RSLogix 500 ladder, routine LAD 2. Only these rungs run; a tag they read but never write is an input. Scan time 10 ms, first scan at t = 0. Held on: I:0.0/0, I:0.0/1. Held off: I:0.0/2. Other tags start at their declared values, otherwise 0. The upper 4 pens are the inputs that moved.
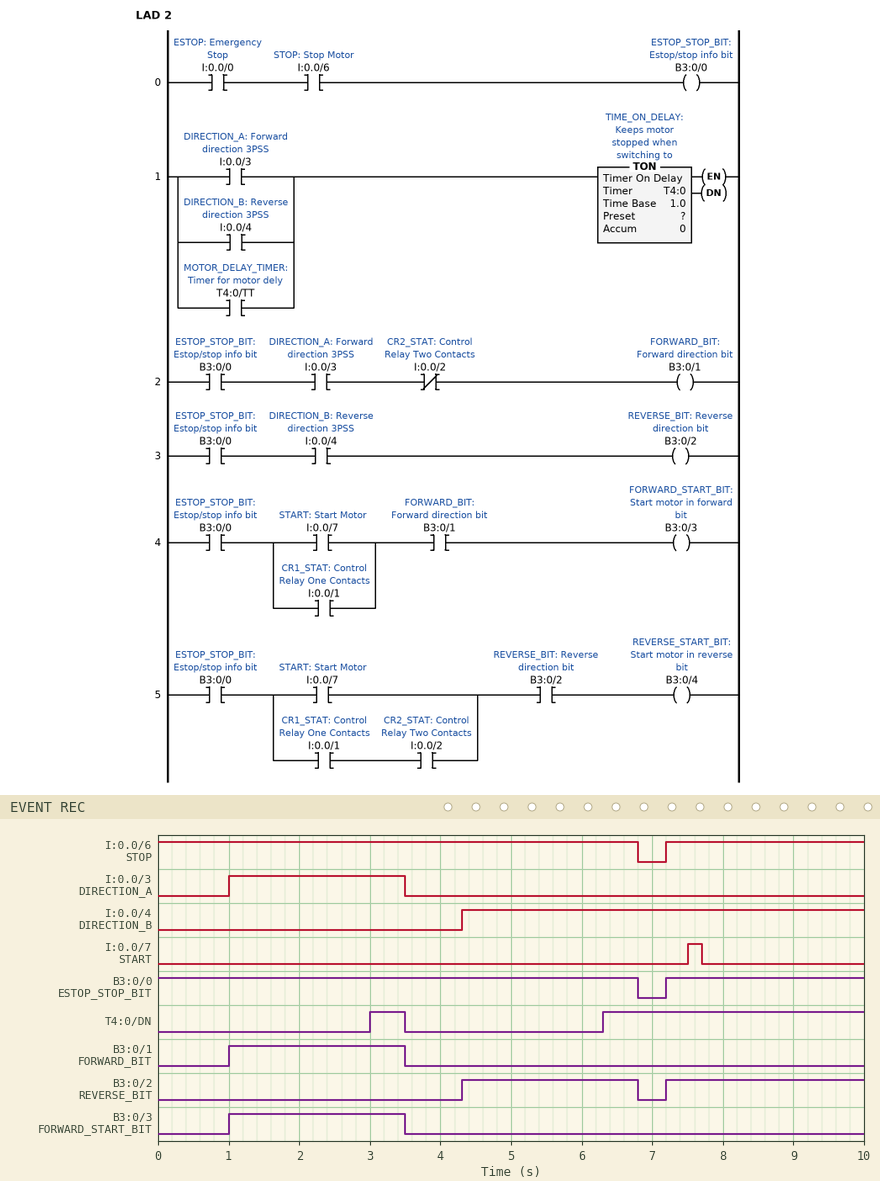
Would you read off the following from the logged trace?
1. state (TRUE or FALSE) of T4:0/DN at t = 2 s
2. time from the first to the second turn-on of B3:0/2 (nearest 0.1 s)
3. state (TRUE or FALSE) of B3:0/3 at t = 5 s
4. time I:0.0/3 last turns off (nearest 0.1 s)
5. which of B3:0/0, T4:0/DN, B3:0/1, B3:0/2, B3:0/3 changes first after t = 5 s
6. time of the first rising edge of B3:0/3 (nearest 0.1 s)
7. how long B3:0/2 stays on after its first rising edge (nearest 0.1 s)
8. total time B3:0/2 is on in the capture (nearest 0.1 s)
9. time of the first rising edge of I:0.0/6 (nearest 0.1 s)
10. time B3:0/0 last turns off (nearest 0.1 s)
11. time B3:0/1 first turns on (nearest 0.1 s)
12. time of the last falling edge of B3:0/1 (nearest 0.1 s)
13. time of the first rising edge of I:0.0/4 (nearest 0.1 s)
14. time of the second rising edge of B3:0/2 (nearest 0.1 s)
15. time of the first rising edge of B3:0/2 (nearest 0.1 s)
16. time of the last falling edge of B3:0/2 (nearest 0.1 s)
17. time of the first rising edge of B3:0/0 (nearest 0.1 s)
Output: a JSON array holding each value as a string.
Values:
["FALSE", "2.9 s", "FALSE", "3.5 s", "T4:0/DN", "1.0 s", "2.5 s", "5.3 s", "7.2 s", "6.8 s", "1.0 s", "3.5 s", "4.3 s", "7.2 s", "4.3 s", "6.8 s", "7.2 s"]
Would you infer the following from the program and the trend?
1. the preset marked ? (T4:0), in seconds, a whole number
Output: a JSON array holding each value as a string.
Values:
["2 s"]
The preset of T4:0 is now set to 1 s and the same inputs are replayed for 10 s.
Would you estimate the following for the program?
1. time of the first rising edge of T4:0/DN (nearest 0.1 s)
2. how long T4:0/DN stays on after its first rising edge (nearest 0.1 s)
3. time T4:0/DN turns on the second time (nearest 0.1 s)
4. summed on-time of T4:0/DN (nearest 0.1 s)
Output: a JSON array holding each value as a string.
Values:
["2.0 s", "1.5 s", "5.3 s", "6.2 s"]
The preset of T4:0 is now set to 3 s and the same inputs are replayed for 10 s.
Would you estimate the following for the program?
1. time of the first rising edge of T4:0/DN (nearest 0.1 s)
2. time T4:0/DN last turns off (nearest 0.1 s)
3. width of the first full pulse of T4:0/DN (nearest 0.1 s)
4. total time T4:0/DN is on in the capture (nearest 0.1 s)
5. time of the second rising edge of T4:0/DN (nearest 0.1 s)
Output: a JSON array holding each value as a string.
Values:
["4.0 s", "4.0 s", "0.0 s", "2.7 s", "7.3 s"]
